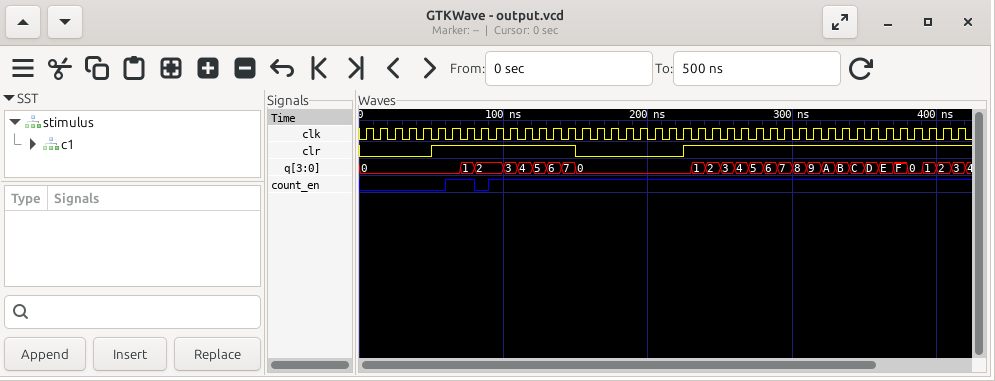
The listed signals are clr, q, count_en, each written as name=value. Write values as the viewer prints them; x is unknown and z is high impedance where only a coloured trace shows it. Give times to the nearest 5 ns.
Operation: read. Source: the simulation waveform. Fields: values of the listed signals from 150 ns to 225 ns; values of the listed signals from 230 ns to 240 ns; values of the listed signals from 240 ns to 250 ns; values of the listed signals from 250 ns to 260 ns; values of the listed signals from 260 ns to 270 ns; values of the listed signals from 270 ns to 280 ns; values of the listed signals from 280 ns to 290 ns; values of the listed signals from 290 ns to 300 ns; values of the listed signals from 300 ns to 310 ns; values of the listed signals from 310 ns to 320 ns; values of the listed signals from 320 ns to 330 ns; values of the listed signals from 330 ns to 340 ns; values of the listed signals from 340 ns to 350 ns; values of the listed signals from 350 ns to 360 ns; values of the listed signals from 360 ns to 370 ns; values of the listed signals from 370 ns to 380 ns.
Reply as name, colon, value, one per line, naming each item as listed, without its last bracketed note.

values of the listed signals from 150 ns to 225 ns: clr=0, q=0, count_en=1
values of the listed signals from 230 ns to 240 ns: clr=1, q=1, count_en=1
values of the listed signals from 240 ns to 250 ns: clr=1, q=2, count_en=1
values of the listed signals from 250 ns to 260 ns: clr=1, q=3, count_en=1
values of the listed signals from 260 ns to 270 ns: clr=1, q=4, count_en=1
values of the listed signals from 270 ns to 280 ns: clr=1, q=5, count_en=1
values of the listed signals from 280 ns to 290 ns: clr=1, q=6, count_en=1
values of the listed signals from 290 ns to 300 ns: clr=1, q=7, count_en=1
values of the listed signals from 300 ns to 310 ns: clr=1, q=8, count_en=1
values of the listed signals from 310 ns to 320 ns: clr=1, q=9, count_en=1
values of the listed signals from 320 ns to 330 ns: clr=1, q=A, count_en=1
values of the listed signals from 330 ns to 340 ns: clr=1, q=B, count_en=1
values of the listed signals from 340 ns to 350 ns: clr=1, q=C, count_en=1
values of the listed signals from 350 ns to 360 ns: clr=1, q=D, count_en=1
values of the listed signals from 360 ns to 370 ns: clr=1, q=E, count_en=1
values of the listed signals from 370 ns to 380 ns: clr=1, q=F, count_en=1
